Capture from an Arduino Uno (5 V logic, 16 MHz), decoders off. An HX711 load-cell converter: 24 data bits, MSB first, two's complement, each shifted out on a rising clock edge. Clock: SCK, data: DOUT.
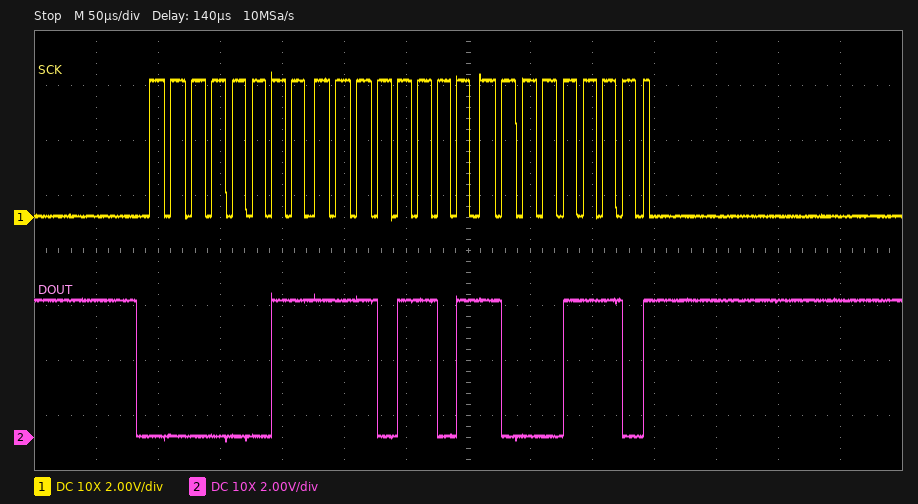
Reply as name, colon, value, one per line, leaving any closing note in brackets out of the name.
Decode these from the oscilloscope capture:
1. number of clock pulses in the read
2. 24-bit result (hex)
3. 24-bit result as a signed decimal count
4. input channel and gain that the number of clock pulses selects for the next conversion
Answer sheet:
number of clock pulses in the read: 25
24-bit result: 0x03ED8E
24-bit result as a signed decimal count: 257422
input channel and gain that the number of clock pulses selects for the next conversion: channel A, gain 128
